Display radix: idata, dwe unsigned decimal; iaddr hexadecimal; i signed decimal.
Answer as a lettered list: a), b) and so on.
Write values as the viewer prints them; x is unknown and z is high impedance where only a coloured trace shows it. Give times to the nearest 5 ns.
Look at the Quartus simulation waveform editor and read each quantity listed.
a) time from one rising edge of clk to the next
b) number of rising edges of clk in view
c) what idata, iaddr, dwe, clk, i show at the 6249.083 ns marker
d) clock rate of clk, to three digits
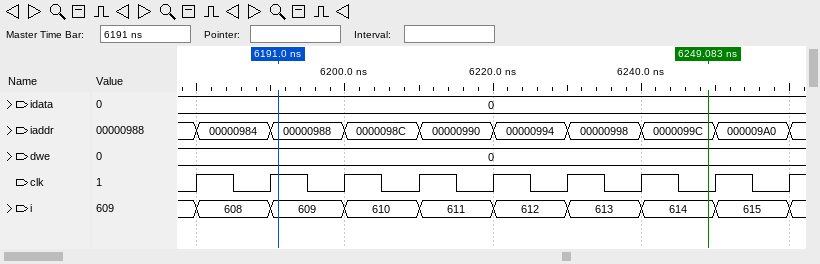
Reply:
a) 10 ns
b) 9
c) idata=0, iaddr=0000099C, dwe=0, clk=0, i=614
d) 100 MHz
